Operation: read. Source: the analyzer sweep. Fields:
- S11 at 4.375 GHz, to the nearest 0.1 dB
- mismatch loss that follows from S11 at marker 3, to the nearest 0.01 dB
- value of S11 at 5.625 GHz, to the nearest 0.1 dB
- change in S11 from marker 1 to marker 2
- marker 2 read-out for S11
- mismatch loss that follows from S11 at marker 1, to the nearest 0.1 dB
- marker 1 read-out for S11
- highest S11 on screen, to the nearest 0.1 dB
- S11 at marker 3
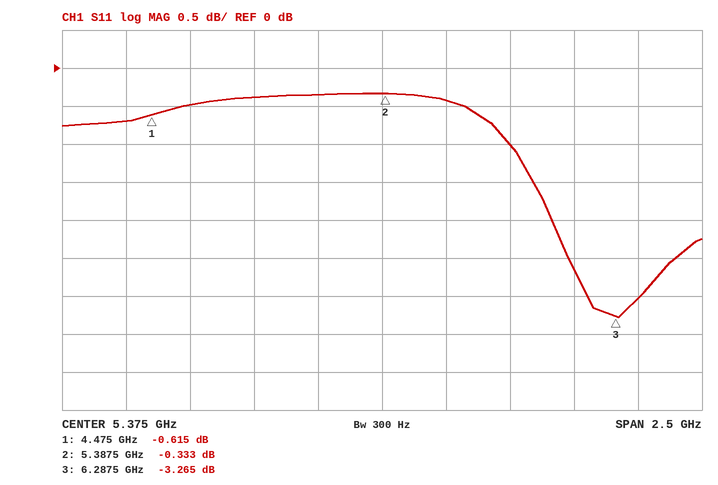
-0.7 dB
2.77 dB
-0.4 dB
0.282 dB
-0.333 dB
8.8 dB
-0.615 dB
-0.3 dB
-3.265 dB
